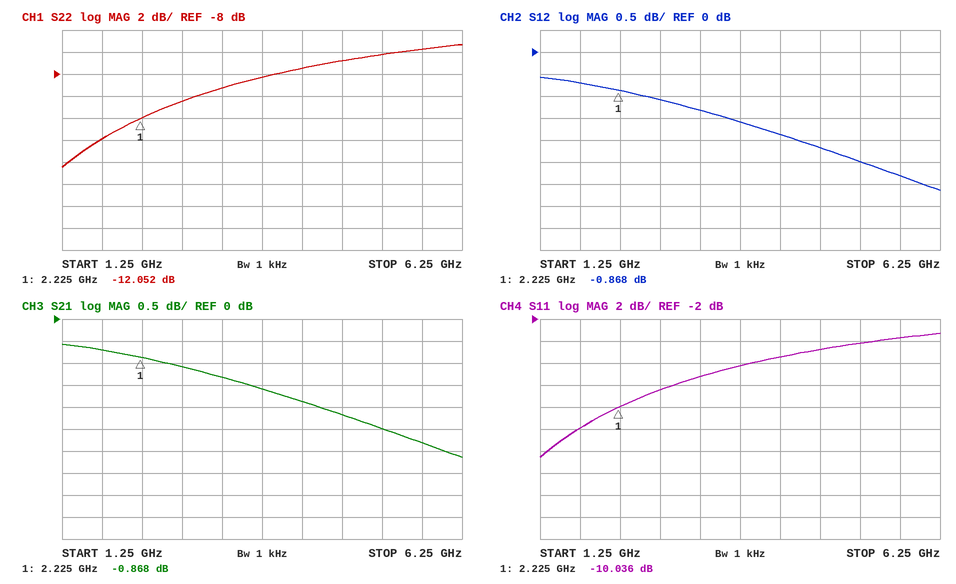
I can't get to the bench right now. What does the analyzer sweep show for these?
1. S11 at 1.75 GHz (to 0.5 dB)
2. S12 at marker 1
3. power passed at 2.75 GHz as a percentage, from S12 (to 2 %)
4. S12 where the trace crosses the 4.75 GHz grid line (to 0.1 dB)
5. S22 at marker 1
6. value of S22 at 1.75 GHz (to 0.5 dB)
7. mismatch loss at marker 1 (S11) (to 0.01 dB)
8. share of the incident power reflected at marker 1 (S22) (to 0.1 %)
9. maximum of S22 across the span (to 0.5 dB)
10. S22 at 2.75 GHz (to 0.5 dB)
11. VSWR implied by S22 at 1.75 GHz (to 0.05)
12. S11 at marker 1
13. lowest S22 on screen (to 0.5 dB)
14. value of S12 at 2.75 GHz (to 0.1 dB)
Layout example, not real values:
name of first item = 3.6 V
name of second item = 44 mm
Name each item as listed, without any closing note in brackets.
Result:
S11 at 1.75 GHz = -12.0 dB
S12 at marker 1 = -0.868 dB
power passed at 2.75 GHz as a percentage, from S12 = 78 %
S12 where the trace crosses the 4.75 GHz grid line = -2.2 dB
S22 at marker 1 = -12.052 dB
value of S22 at 1.75 GHz = -14.0 dB
mismatch loss at marker 1 (S11) = 0.45 dB
share of the incident power reflected at marker 1 (S22) = 6.2 %
maximum of S22 across the span = -5.5 dB
S22 at 2.75 GHz = -10.5 dB
VSWR implied by S22 at 1.75 GHz = 1.50
S11 at marker 1 = -10.036 dB
lowest S22 on screen = -16.5 dB
value of S12 at 2.75 GHz = -1.1 dB
